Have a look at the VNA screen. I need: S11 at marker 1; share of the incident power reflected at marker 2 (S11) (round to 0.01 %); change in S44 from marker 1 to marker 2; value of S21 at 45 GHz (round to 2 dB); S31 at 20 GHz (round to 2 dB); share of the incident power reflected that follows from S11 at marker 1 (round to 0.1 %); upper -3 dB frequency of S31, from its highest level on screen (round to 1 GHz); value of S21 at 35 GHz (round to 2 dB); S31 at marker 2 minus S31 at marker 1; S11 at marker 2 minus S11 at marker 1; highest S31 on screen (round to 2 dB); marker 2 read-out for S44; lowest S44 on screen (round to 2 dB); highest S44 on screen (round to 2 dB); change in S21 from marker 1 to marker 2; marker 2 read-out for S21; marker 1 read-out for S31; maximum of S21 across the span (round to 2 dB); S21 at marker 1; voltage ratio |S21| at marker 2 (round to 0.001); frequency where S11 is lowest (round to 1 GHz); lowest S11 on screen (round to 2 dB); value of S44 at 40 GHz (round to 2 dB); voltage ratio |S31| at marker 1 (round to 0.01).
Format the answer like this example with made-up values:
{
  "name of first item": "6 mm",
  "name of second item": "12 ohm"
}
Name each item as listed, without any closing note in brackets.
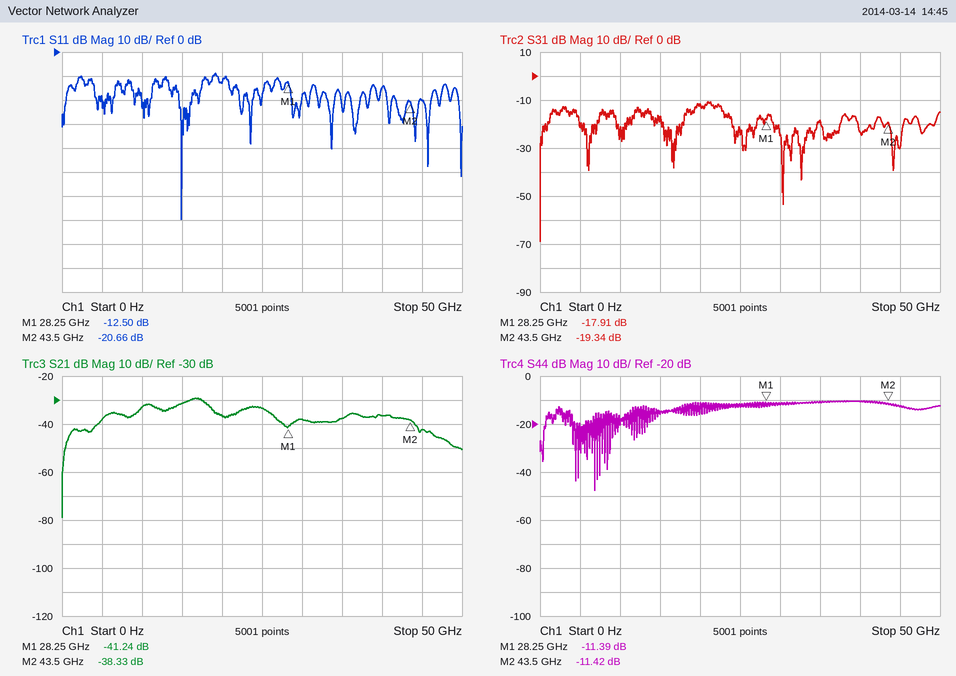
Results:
{
  "S11 at marker 1": "-12.50 dB",
  "share of the incident power reflected at marker 2 (S11)": "0.86 %",
  "change in S44 from marker 1 to marker 2": "-0.03 dB",
  "value of S21 at 45 GHz": "-42 dB",
  "S31 at 20 GHz": "-12 dB",
  "share of the incident power reflected that follows from S11 at marker 1": "5.6 %",
  "upper -3 dB frequency of S31, from its highest level on screen": "23 GHz",
  "value of S21 at 35 GHz": "-38 dB",
  "S31 at marker 2 minus S31 at marker 1": "-1.43 dB",
  "S11 at marker 2 minus S11 at marker 1": "-8.16 dB",
  "highest S31 on screen": "-10 dB",
  "marker 2 read-out for S44": "-11.42 dB",
  "lowest S44 on screen": "-48 dB",
  "highest S44 on screen": "-10 dB",
  "change in S21 from marker 1 to marker 2": "2.91 dB",
  "marker 2 read-out for S21": "-38.33 dB",
  "marker 1 read-out for S31": "-17.91 dB",
  "maximum of S21 across the span": "-30 dB",
  "S21 at marker 1": "-41.24 dB",
  "voltage ratio |S21| at marker 2": "0.012",
  "frequency where S11 is lowest": "15 GHz",
  "lowest S11 on screen": "-70 dB",
  "value of S44 at 40 GHz": "-10 dB",
  "voltage ratio |S31| at marker 1": "0.13"
}
